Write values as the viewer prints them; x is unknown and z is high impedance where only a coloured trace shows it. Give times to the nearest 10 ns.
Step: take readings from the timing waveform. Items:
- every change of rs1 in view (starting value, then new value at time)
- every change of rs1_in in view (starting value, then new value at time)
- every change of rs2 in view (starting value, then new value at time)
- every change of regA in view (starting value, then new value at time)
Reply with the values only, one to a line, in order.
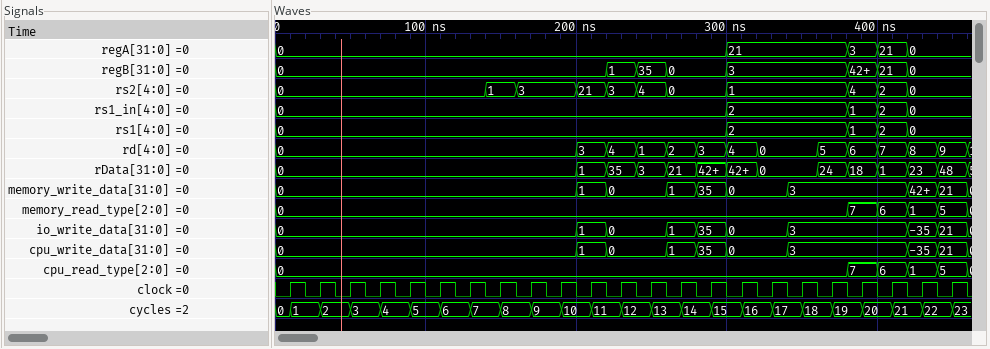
0, 2 at 300 ns, 1 at 380 ns, 2 at 400 ns, 0 at 420 ns
0, 2 at 300 ns, 1 at 380 ns, 2 at 400 ns, 0 at 420 ns
0, 1 at 140 ns, 3 at 160 ns, 21 at 200 ns, 3 at 220 ns, 4 at 240 ns, 0 at 260 ns, 1 at 300 ns, 4 at 380 ns, 2 at 400 ns, 0 at 420 ns
0, 21 at 300 ns, 3 at 380 ns, 21 at 400 ns, 0 at 420 ns
